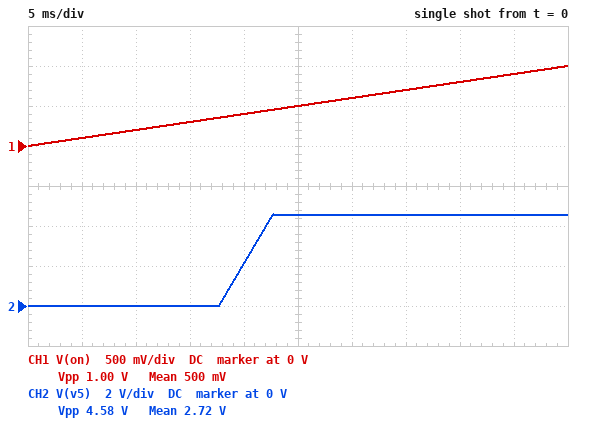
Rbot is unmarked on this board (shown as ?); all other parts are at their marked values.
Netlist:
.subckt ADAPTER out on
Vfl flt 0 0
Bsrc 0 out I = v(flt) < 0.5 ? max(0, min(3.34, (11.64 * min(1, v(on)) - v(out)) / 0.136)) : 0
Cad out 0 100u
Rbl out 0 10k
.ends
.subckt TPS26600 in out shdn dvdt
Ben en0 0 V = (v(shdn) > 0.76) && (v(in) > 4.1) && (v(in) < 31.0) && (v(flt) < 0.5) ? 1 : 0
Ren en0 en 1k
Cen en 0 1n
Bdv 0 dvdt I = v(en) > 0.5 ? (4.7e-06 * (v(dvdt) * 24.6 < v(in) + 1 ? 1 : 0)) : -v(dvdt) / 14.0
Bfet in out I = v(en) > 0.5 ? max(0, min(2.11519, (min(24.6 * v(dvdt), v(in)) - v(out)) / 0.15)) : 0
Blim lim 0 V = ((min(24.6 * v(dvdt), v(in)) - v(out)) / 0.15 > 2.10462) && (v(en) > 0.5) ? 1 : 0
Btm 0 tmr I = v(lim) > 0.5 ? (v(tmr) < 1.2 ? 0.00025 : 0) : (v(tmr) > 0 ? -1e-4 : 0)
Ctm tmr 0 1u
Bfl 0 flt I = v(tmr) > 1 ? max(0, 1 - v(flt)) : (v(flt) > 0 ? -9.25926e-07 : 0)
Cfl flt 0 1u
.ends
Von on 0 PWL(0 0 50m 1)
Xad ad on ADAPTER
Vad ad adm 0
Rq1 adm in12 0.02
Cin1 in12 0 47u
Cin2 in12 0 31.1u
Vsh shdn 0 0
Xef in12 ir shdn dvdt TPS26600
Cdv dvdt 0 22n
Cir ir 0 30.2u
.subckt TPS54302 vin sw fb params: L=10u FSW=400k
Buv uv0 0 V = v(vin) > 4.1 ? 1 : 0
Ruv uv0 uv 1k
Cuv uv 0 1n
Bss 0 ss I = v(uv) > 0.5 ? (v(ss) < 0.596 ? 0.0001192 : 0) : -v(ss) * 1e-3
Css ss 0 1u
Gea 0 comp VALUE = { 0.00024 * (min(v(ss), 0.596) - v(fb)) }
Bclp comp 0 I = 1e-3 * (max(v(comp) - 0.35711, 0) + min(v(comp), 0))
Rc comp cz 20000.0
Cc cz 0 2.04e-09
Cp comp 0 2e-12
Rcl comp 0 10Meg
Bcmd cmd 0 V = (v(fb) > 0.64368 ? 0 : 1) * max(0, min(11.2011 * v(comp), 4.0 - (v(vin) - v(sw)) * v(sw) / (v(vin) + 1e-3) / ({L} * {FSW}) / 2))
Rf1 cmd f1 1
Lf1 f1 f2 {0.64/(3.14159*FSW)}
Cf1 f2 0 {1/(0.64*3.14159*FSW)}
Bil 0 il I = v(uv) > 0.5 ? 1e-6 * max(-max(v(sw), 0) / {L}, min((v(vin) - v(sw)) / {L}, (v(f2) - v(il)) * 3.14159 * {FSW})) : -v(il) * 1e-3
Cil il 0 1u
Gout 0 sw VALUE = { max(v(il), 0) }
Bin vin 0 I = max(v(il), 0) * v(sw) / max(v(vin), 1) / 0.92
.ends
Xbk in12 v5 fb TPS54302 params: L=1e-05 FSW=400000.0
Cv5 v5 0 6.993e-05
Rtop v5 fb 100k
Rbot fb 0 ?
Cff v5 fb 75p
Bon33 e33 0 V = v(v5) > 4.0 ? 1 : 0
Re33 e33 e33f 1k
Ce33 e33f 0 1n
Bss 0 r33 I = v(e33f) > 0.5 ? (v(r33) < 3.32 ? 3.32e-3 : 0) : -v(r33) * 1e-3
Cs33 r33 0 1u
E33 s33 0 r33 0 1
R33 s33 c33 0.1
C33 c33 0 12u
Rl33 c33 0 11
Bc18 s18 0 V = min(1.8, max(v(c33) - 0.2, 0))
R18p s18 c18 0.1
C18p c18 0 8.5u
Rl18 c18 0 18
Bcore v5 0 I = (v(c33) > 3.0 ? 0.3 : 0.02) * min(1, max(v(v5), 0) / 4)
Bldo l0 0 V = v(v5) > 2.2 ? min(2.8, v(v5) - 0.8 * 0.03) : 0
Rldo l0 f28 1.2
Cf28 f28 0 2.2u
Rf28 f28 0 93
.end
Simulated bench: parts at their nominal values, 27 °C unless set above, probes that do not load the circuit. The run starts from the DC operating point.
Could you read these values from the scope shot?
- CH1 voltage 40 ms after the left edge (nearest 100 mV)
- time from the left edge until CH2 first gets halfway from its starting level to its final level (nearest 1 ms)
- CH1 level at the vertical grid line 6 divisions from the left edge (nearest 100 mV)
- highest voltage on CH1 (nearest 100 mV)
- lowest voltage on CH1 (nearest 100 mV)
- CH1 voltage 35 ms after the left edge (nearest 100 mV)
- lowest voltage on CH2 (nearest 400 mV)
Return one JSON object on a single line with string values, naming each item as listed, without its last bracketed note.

{"CH1 voltage 40 ms after the left edge": "800 mV", "time from the left edge until CH2 first gets halfway from its starting level to its final level": "20 ms", "CH1 level at the vertical grid line 6 divisions from the left edge": "600 mV", "highest voltage on CH1": "1.0 V", "lowest voltage on CH1": "0 V", "CH1 voltage 35 ms after the left edge": "700 mV", "lowest voltage on CH2": "0 V"}
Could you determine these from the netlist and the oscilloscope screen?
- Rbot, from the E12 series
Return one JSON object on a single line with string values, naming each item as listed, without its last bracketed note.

{"Rbot, from the E12 series": "15 kΩ"}
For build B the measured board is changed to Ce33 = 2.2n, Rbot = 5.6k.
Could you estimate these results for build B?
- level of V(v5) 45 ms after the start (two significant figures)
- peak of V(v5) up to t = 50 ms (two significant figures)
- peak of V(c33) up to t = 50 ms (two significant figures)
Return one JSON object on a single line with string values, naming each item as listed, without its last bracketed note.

{"level of V(v5) 45 ms after the start": "10 V", "peak of V(v5) up to t = 50 ms": "11 V", "peak of V(c33) up to t = 50 ms": "3.3 V"}
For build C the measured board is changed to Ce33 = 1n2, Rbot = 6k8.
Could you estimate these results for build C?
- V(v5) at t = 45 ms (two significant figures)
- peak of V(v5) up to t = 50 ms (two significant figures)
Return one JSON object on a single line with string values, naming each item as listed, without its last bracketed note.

{"V(v5) at t = 45 ms": "9.4 V", "peak of V(v5) up to t = 50 ms": "9.5 V"}
